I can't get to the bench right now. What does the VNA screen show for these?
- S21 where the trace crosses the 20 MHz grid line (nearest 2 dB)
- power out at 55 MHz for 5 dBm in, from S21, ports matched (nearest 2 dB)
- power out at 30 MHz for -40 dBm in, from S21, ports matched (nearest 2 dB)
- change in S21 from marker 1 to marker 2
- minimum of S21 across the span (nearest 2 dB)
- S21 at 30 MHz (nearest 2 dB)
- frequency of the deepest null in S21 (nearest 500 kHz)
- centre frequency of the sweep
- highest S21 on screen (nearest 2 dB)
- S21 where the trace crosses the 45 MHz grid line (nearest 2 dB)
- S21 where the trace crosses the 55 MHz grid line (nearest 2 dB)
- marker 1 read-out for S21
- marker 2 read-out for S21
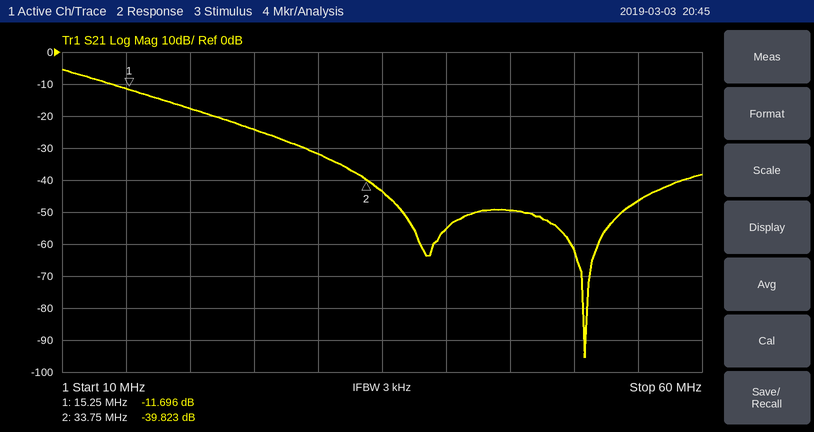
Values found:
-18 dB
-42 dBm
-72 dBm
-28.127 dB
-96 dB
-32 dB
51.0 MHz
35 MHz
-6 dB
-50 dB
-46 dB
-11.696 dB
-39.823 dB
